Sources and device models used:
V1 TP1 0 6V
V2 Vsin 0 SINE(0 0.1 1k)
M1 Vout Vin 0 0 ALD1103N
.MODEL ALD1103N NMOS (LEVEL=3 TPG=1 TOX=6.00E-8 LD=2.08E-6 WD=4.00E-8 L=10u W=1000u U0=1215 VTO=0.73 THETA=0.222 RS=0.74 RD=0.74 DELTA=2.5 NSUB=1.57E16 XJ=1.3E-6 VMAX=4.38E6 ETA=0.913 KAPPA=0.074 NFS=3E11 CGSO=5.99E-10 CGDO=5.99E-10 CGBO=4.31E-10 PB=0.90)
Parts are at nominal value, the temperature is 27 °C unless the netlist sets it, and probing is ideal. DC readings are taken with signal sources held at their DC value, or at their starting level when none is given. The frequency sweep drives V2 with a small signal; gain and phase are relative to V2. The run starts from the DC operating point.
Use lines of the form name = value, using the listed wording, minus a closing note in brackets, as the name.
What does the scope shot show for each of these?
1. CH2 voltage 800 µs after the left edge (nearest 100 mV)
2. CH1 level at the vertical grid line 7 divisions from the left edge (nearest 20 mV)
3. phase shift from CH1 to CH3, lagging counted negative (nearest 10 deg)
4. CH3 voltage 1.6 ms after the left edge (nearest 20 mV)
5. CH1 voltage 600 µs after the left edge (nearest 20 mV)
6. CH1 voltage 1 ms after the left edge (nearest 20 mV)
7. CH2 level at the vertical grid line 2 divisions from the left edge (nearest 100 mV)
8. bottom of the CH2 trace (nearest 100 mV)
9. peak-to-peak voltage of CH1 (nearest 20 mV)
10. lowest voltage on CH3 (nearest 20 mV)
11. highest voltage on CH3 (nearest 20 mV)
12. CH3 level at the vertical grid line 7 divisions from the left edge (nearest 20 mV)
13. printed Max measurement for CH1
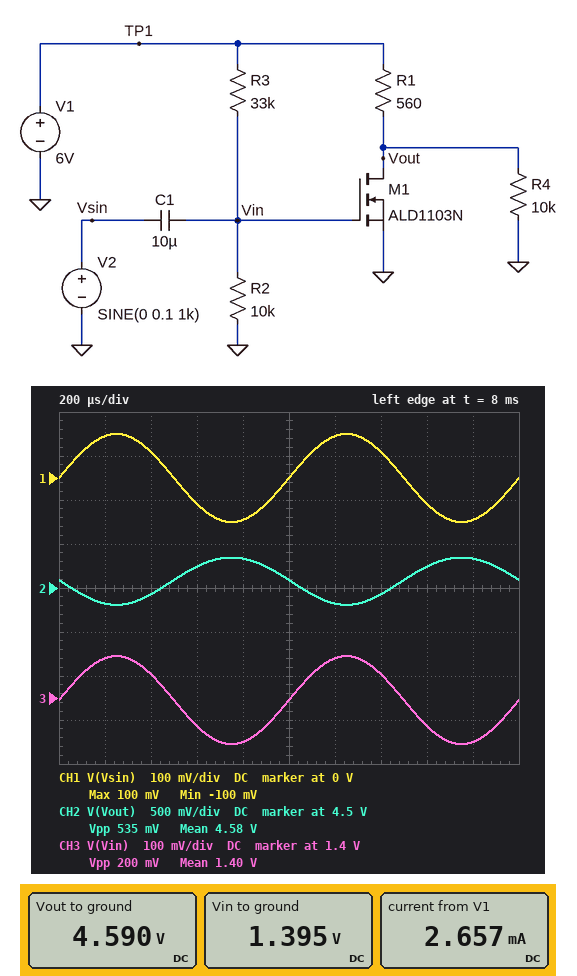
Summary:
CH2 voltage 800 µs after the left edge = 4.8 V
CH1 level at the vertical grid line 7 divisions from the left edge = 60 mV
phase shift from CH1 to CH3, lagging counted negative = 0 deg
CH3 voltage 1.6 ms after the left edge = 1.34 V
CH1 voltage 600 µs after the left edge = -60 mV
CH1 voltage 1 ms after the left edge = 0 V
CH2 level at the vertical grid line 2 divisions from the left edge = 4.4 V
bottom of the CH2 trace = 4.3 V
peak-to-peak voltage of CH1 = 200 mV
lowest voltage on CH3 = 1.30 V
highest voltage on CH3 = 1.50 V
CH3 level at the vertical grid line 7 divisions from the left edge = 1.46 V
printed Max measurement for CH1 = 100 mV
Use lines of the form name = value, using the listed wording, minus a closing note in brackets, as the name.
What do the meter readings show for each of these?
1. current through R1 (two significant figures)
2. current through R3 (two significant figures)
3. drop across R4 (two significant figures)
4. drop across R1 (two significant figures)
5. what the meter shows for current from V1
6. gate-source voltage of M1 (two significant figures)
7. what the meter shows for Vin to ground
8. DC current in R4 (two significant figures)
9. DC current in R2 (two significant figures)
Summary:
current through R1 = 2.5 mA
current through R3 = 140 µA
drop across R4 = 4.6 V
drop across R1 = 1.4 V
what the meter shows for current from V1 = 2.657 mA
gate-source voltage of M1 = 1.4 V
what the meter shows for Vin to ground = 1.395 V
DC current in R4 = 460 µA
DC current in R2 = 140 µA
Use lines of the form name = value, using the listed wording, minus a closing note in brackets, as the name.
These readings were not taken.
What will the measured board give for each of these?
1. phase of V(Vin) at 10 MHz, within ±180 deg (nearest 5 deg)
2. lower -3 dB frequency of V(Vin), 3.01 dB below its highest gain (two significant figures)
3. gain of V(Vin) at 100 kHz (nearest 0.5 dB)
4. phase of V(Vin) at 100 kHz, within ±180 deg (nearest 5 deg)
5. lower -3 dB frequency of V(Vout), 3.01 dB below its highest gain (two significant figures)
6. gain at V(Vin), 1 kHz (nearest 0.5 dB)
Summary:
phase of V(Vin) at 10 MHz, within ±180 deg = 0 deg
lower -3 dB frequency of V(Vin), 3.01 dB below its highest gain = 2.1 Hz
gain of V(Vin) at 100 kHz = 0 dB
phase of V(Vin) at 100 kHz, within ±180 deg = 0 deg
lower -3 dB frequency of V(Vout), 3.01 dB below its highest gain = 2.1 Hz
gain at V(Vin), 1 kHz = 0 dB
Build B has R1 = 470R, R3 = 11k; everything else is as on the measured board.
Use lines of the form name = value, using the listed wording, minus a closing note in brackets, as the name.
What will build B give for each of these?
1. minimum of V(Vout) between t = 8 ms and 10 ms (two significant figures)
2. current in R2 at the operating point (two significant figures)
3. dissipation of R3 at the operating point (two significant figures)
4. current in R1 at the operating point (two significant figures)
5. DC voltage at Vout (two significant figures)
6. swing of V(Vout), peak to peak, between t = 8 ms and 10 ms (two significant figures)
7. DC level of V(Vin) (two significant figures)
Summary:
minimum of V(Vout) between t = 8 ms and 10 ms = 820 mV
current in R2 at the operating point = 290 µA
dissipation of R3 at the operating point = 900 µW
current in R1 at the operating point = 11 mA
DC voltage at Vout = 860 mV
swing of V(Vout), peak to peak, between t = 8 ms and 10 ms = 100 mV
DC level of V(Vin) = 2.9 V
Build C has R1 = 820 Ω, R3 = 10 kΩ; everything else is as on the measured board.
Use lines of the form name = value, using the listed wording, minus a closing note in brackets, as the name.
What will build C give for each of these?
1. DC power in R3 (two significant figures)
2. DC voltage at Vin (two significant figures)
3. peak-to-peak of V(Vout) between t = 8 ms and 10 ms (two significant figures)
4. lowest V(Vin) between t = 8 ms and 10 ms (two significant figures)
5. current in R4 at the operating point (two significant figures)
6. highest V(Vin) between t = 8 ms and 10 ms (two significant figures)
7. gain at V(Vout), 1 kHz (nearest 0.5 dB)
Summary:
DC power in R3 = 900 µW
DC voltage at Vin = 3.0 V
peak-to-peak of V(Vout) between t = 8 ms and 10 ms = 31 mV
lowest V(Vin) between t = 8 ms and 10 ms = 2.9 V
current in R4 at the operating point = 43 µA
highest V(Vin) between t = 8 ms and 10 ms = 3.1 V
gain at V(Vout), 1 kHz = -16.0 dB
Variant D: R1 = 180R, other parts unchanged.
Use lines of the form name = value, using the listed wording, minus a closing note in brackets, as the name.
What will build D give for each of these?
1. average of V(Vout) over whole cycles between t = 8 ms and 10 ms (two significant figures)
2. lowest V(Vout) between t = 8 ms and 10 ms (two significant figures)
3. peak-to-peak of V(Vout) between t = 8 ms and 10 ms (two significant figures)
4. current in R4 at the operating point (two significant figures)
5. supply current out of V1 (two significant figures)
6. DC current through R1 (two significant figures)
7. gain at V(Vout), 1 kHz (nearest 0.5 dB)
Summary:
average of V(Vout) over whole cycles between t = 8 ms and 10 ms = 5.5 V
lowest V(Vout) between t = 8 ms and 10 ms = 5.4 V
peak-to-peak of V(Vout) between t = 8 ms and 10 ms = 180 mV
current in R4 at the operating point = 550 µA
supply current out of V1 = 2.8 mA
DC current through R1 = 2.6 mA
gain at V(Vout), 1 kHz = -1.0 dB
